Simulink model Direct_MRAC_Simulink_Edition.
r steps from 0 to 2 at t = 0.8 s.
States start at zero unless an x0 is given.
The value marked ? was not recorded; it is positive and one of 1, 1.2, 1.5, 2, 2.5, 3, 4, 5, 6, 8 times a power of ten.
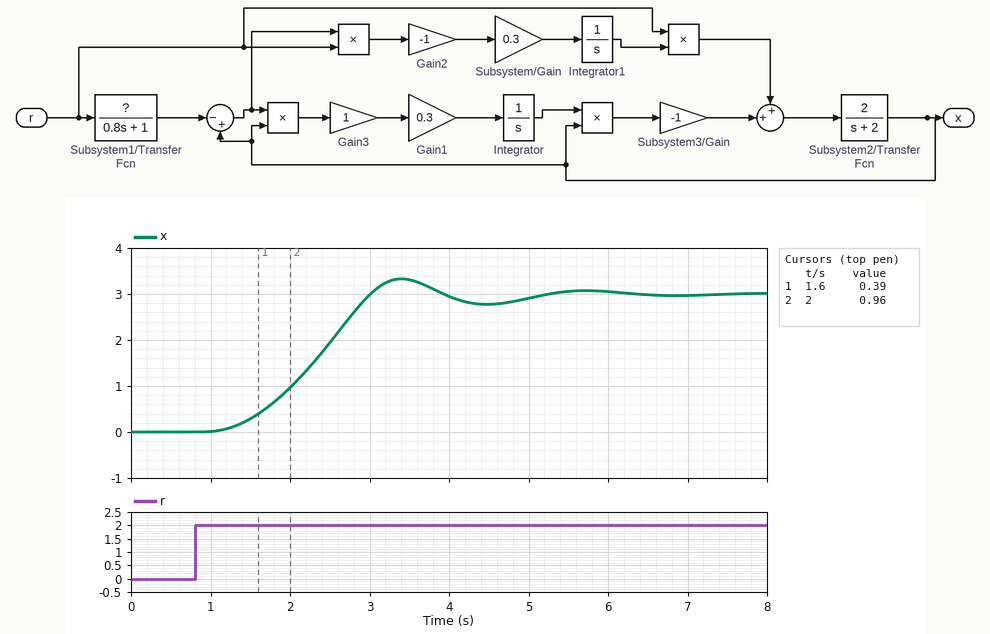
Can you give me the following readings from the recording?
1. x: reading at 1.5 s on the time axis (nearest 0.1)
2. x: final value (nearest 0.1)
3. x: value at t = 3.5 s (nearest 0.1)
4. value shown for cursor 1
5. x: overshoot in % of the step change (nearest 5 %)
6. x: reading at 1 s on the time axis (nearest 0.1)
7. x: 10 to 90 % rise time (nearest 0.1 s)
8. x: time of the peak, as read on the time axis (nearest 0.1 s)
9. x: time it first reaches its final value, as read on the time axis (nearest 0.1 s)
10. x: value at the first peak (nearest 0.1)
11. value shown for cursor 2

0.3
3.0
3.3
0.39
10 %
0.0
1.3 s
3.4 s
3.0 s
3.3
0.96
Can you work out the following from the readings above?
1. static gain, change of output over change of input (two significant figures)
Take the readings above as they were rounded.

1.5
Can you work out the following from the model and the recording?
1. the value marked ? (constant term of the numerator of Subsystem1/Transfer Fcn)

1.5
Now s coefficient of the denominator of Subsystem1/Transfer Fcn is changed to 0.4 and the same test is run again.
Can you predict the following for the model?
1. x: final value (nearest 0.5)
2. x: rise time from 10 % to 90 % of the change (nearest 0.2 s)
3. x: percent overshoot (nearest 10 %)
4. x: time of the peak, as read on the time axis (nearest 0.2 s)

3.0
1.0 s
20 %
3.0 s
